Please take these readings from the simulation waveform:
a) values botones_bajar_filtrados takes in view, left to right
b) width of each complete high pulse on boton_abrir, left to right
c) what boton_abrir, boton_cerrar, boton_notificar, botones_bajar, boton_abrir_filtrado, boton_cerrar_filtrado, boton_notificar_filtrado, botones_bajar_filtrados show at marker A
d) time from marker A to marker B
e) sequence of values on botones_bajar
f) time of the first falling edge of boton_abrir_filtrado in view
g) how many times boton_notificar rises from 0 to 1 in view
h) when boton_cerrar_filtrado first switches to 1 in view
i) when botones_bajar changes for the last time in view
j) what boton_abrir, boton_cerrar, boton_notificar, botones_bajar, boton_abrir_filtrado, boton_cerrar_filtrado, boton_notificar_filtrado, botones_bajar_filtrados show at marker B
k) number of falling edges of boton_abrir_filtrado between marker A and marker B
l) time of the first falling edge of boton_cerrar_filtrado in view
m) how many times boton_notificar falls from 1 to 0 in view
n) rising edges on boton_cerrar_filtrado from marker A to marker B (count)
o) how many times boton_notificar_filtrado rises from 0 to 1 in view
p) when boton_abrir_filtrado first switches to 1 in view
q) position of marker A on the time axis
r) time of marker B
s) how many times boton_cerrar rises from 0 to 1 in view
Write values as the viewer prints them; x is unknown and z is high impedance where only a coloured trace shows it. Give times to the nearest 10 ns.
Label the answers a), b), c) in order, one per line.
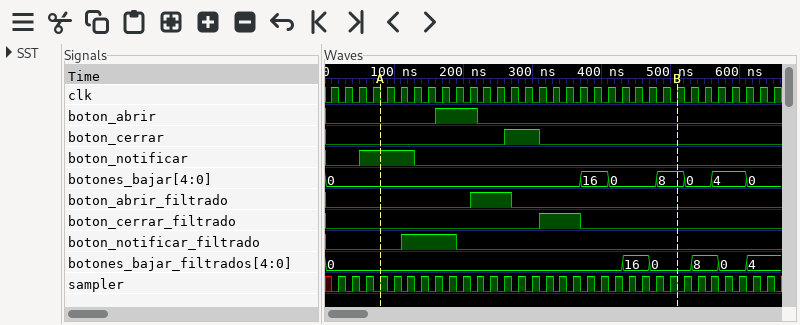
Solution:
a) 0, 16, 0, 8, 0, 4
b) 60 ns
c) boton_abrir=0, boton_cerrar=0, boton_notificar=1, botones_bajar=0, boton_abrir_filtrado=0, boton_cerrar_filtrado=0, boton_notificar_filtrado=0, botones_bajar_filtrados=0
d) 430 ns
e) 0, 16, 0, 8, 0, 4, 0
f) 270 ns
g) 1
h) 310 ns
i) 610 ns
j) boton_abrir=0, boton_cerrar=0, boton_notificar=0, botones_bajar=8, boton_abrir_filtrado=0, boton_cerrar_filtrado=0, boton_notificar_filtrado=0, botones_bajar_filtrados=0
k) 1
l) 370 ns
m) 1
n) 1
o) 1
p) 210 ns
q) 80 ns
r) 510 ns
s) 1
